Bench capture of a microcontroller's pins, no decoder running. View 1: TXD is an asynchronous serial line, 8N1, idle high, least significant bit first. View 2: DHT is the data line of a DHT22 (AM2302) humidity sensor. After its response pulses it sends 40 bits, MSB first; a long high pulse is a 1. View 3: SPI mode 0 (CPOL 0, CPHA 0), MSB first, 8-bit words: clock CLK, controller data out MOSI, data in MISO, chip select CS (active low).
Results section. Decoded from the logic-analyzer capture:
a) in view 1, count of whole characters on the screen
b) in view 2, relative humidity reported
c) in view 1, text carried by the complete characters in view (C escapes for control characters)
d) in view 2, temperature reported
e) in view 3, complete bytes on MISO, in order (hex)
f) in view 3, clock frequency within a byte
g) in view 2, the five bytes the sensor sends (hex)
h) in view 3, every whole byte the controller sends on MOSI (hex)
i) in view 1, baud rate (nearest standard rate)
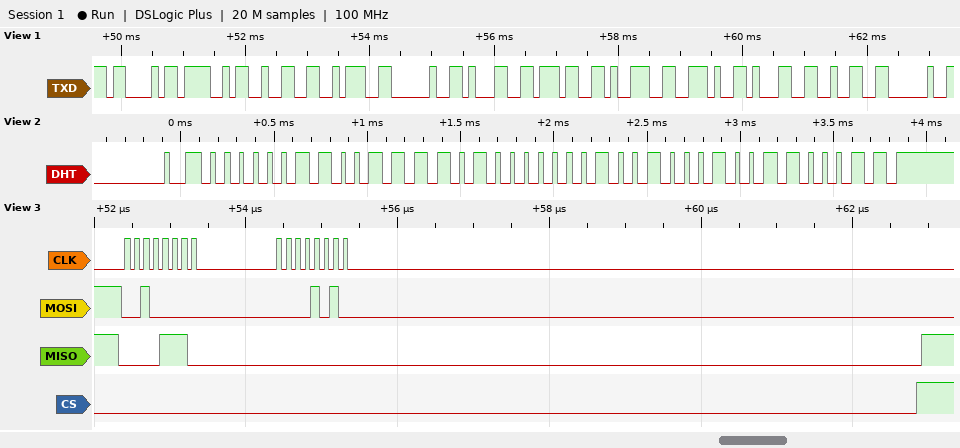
12
82.9 %
"CO2: 179.12 "
29.0 °C
0E 00
8 MHz
03 3D 01 22 63
20 0A
9600 baud
